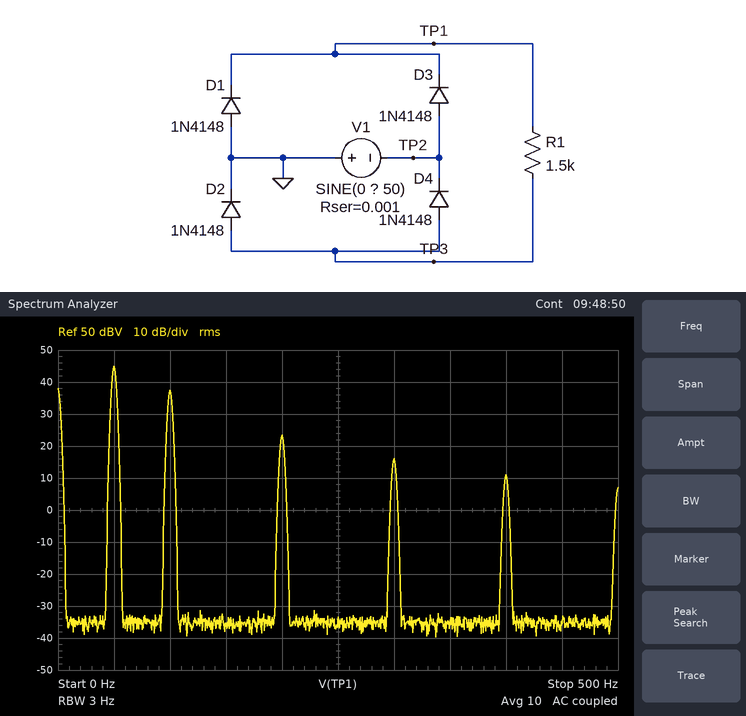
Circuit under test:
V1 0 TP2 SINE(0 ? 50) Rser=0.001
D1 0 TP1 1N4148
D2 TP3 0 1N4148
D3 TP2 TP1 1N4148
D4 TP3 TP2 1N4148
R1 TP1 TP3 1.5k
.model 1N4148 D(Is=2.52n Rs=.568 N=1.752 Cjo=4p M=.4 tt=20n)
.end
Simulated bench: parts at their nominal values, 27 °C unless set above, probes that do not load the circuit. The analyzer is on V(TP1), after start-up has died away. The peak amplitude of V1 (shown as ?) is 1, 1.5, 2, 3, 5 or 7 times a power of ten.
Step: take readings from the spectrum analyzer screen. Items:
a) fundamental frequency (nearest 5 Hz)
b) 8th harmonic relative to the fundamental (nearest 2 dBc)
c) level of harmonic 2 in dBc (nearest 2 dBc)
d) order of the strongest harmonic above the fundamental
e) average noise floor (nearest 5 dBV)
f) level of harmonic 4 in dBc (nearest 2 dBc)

50 Hz
-34 dBc
-8 dBc
2
-35 dBV
-22 dBc
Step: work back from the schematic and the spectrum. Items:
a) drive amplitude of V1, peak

500 V
